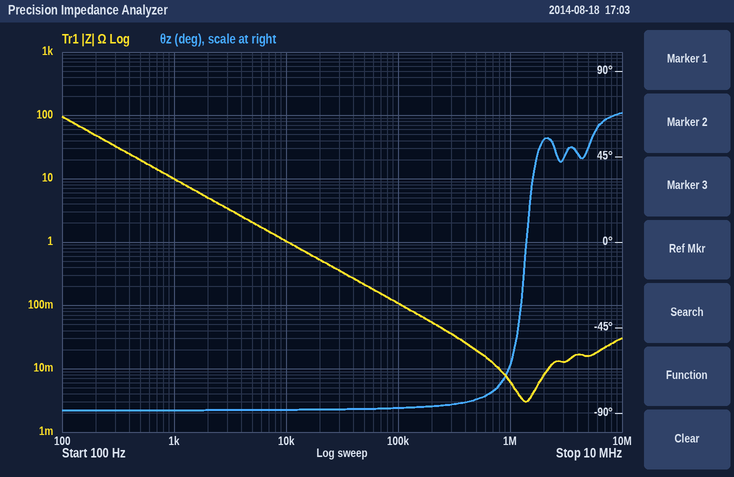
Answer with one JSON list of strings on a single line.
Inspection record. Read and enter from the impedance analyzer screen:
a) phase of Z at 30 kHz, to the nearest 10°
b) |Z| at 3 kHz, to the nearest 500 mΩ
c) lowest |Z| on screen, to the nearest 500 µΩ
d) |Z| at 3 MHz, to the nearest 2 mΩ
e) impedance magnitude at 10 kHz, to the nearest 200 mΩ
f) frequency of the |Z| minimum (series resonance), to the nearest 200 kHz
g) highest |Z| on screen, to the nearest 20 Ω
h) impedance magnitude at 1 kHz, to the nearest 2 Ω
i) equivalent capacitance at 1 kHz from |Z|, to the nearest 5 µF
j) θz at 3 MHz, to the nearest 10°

["-90°", "3.5 Ω", "3.0 mΩ", "12 mΩ", "1.0 Ω", "1.4 MHz", "100 Ω", "10 Ω", "15 µF", "40°"]
